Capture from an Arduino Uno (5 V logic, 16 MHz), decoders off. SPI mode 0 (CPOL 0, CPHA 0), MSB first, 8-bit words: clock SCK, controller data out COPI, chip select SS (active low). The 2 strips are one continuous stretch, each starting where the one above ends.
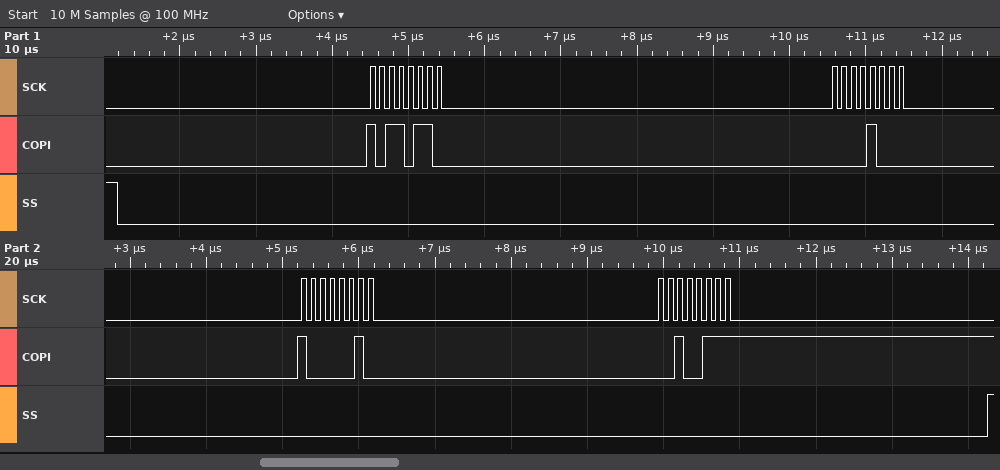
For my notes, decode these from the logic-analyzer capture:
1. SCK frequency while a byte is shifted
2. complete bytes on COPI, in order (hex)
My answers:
8 MHz
B6 08 82 27
